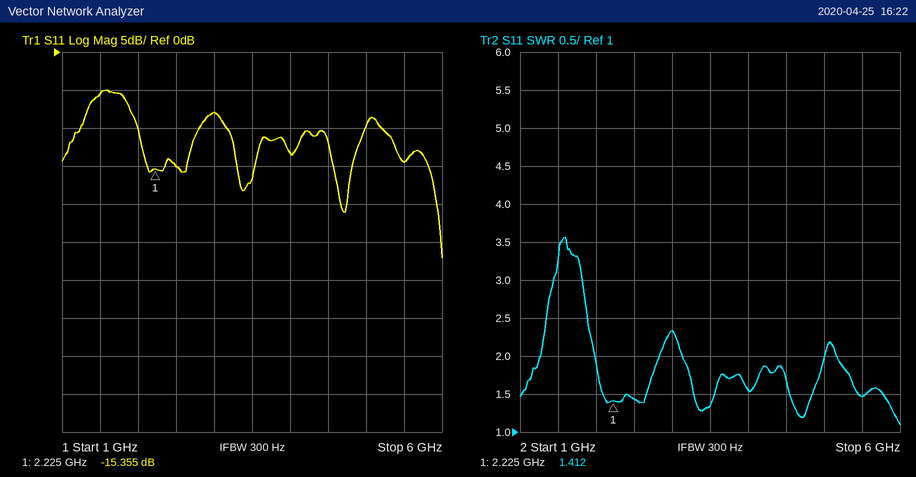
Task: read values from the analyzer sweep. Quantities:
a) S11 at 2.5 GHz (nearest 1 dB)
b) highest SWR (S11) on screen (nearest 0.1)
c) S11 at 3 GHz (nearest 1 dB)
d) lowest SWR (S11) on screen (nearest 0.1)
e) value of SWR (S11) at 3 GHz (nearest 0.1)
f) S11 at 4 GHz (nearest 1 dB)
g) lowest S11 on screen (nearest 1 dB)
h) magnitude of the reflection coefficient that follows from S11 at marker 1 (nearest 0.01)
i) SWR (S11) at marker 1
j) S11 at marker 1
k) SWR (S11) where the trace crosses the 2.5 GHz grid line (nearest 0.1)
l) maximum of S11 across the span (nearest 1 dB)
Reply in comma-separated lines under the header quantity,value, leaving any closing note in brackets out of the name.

quantity,value
S11 at 2.5 GHz,-15 dB
highest SWR (S11) on screen,3.6
S11 at 3 GHz,-8 dB
lowest SWR (S11) on screen,1.1
value of SWR (S11) at 3 GHz,2.3
S11 at 4 GHz,-13 dB
lowest S11 on screen,-27 dB
magnitude of the reflection coefficient that follows from S11 at marker 1,0.17
SWR (S11) at marker 1,1.412
S11 at marker 1,-15.355 dB
SWR (S11) where the trace crosses the 2.5 GHz grid line,1.4
maximum of S11 across the span,-5 dB
